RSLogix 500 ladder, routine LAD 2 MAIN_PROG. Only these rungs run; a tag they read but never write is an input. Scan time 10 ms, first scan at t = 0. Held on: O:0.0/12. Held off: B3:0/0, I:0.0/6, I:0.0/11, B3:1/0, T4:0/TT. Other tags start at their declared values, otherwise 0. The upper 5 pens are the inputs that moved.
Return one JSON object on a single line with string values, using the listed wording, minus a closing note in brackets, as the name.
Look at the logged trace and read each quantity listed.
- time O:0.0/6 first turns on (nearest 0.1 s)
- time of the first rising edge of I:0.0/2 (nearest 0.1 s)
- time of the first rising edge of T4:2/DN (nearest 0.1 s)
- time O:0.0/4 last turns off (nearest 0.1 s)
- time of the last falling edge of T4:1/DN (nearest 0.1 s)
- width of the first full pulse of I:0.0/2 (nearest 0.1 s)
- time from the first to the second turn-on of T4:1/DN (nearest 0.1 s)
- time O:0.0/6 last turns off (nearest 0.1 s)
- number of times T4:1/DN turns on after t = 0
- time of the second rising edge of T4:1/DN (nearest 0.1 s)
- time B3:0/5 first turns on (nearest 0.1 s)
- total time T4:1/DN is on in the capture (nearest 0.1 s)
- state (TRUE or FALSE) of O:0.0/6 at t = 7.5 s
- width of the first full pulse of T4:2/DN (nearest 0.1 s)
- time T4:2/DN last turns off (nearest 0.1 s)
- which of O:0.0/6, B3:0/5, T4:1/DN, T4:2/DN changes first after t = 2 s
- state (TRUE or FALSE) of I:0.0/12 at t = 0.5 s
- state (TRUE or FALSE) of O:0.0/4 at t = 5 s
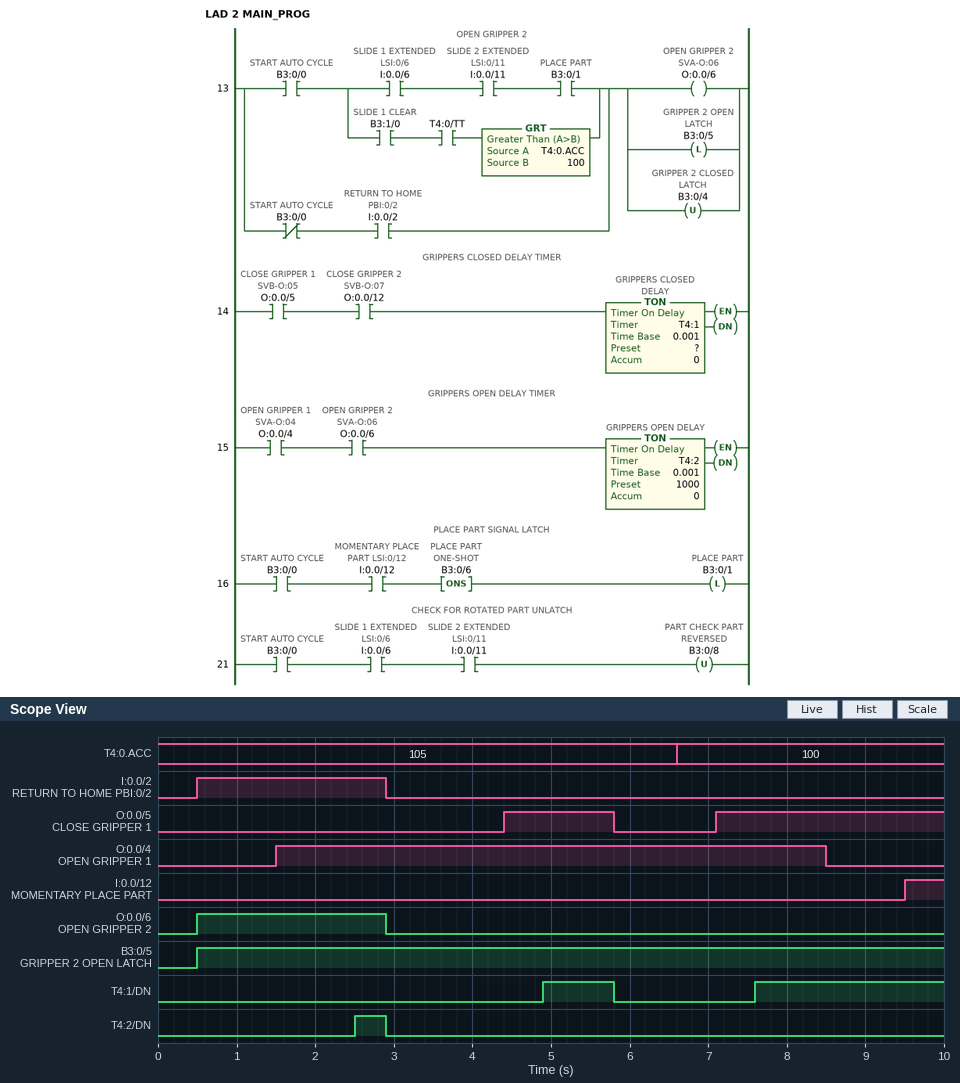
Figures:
{"time O:0.0/6 first turns on": "0.5 s", "time of the first rising edge of I:0.0/2": "0.5 s", "time of the first rising edge of T4:2/DN": "2.5 s", "time O:0.0/4 last turns off": "8.5 s", "time of the last falling edge of T4:1/DN": "5.8 s", "width of the first full pulse of I:0.0/2": "2.4 s", "time from the first to the second turn-on of T4:1/DN": "2.7 s", "time O:0.0/6 last turns off": "2.9 s", "number of times T4:1/DN turns on after t = 0": "2", "time of the second rising edge of T4:1/DN": "7.6 s", "time B3:0/5 first turns on": "0.5 s", "total time T4:1/DN is on in the capture": "3.3 s", "state (TRUE or FALSE) of O:0.0/6 at t = 7.5 s": "FALSE", "width of the first full pulse of T4:2/DN": "0.4 s", "time T4:2/DN last turns off": "2.9 s", "which of O:0.0/6, B3:0/5, T4:1/DN, T4:2/DN changes first after t = 2 s": "T4:2/DN", "state (TRUE or FALSE) of I:0.0/12 at t = 0.5 s": "FALSE", "state (TRUE or FALSE) of O:0.0/4 at t = 5 s": "TRUE"}
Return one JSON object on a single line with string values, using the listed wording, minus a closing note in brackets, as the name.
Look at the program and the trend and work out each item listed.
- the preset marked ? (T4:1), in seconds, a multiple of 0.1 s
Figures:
{"the preset marked ? (T4:1), in seconds, a multiple of 0.1 s": "0.5 s"}
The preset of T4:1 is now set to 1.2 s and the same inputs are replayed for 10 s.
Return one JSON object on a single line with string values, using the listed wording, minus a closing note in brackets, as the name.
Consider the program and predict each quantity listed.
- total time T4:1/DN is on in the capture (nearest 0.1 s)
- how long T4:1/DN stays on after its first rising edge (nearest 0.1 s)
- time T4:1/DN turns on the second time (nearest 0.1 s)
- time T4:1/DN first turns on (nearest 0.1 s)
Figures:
{"total time T4:1/DN is on in the capture": "1.9 s", "how long T4:1/DN stays on after its first rising edge": "0.2 s", "time T4:1/DN turns on the second time": "8.3 s", "time T4:1/DN first turns on": "5.6 s"}
